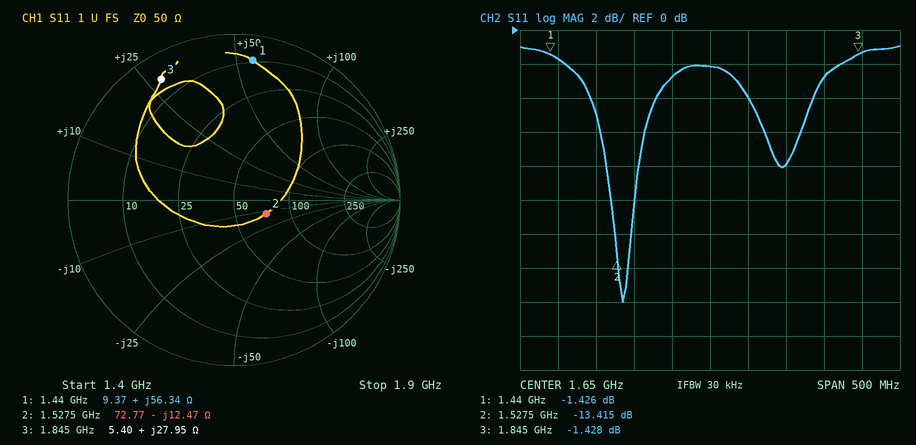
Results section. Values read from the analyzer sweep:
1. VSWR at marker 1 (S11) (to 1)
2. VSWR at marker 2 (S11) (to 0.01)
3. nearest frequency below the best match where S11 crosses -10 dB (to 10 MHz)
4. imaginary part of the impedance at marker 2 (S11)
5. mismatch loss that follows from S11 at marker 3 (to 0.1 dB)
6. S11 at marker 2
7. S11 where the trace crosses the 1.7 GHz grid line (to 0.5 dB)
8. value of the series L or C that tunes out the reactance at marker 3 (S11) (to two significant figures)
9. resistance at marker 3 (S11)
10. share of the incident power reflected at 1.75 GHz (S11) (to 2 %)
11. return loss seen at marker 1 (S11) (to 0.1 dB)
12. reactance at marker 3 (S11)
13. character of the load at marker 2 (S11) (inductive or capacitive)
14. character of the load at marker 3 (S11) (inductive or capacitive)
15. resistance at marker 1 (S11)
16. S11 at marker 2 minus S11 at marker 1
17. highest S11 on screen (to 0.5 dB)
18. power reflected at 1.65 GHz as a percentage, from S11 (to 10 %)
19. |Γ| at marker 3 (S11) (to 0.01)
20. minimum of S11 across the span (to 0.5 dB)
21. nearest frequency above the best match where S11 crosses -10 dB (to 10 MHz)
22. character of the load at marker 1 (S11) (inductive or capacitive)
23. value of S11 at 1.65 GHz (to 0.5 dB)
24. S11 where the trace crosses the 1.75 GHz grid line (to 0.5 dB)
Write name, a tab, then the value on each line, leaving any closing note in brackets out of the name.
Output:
VSWR at marker 1 (S11)	12
VSWR at marker 2 (S11)	1.53
nearest frequency below the best match where S11 crosses -10 dB	1.52 GHz
imaginary part of the impedance at marker 2	-12.47 Ω
mismatch loss that follows from S11 at marker 3	5.5 dB
S11 at marker 2	-13.415 dB
S11 where the trace crosses the 1.7 GHz grid line	-4.0 dB
value of the series L or C that tunes out the reactance at marker 3 (S11)	3.1 pF
resistance at marker 3	5.40 Ω
share of the incident power reflected at 1.75 GHz (S11)	16 %
return loss seen at marker 1 (S11)	1.4 dB
reactance at marker 3	+27.95 Ω
character of the load at marker 2 (S11)	capacitive
character of the load at marker 3 (S11)	inductive
resistance at marker 1	9.37 Ω
S11 at marker 2 minus S11 at marker 1	-11.989 dB
highest S11 on screen	-1.0 dB
power reflected at 1.65 GHz as a percentage, from S11	60 %
|Γ| at marker 3 (S11)	0.85
minimum of S11 across the span	-16.0 dB
nearest frequency above the best match where S11 crosses -10 dB	1.55 GHz
character of the load at marker 1 (S11)	inductive
value of S11 at 1.65 GHz	-2.0 dB
S11 where the trace crosses the 1.75 GHz grid line	-8.0 dB
